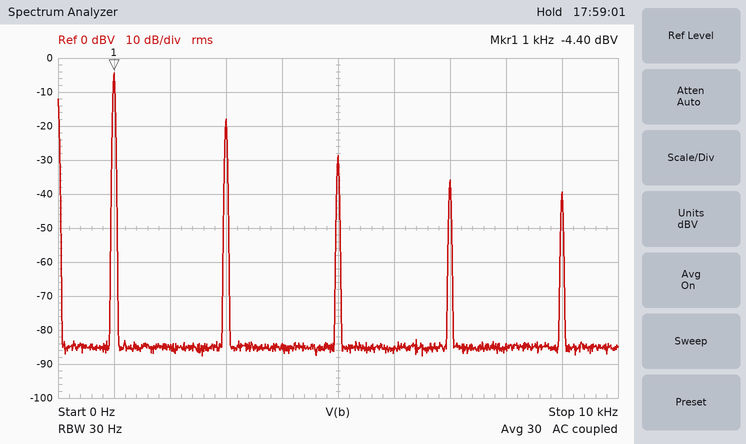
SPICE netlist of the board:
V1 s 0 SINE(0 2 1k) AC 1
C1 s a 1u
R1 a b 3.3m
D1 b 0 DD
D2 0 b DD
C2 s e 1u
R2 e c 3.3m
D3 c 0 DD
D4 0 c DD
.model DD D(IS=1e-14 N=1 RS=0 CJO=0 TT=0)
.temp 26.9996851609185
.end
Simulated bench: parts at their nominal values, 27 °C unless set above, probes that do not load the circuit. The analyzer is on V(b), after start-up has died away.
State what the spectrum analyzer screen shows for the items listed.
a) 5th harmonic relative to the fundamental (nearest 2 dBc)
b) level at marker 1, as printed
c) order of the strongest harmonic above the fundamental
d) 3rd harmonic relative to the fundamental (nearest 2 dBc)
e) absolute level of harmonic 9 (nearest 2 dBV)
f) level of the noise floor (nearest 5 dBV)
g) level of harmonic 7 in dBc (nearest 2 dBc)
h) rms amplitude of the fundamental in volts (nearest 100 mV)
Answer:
-24 dBc
-4.40 dBV
3
-14 dBc
-40 dBV
-85 dBV
-32 dBc
600 mV
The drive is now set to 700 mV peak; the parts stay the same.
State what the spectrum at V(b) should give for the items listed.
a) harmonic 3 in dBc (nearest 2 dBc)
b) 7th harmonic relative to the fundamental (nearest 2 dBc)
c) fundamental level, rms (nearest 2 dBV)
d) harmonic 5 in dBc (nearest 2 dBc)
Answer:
-28 dBc
-44 dBc
-6 dBV
-36 dBc
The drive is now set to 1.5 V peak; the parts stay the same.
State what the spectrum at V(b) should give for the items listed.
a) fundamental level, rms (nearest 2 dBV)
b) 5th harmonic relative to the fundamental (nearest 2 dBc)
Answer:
-4 dBV
-28 dBc
